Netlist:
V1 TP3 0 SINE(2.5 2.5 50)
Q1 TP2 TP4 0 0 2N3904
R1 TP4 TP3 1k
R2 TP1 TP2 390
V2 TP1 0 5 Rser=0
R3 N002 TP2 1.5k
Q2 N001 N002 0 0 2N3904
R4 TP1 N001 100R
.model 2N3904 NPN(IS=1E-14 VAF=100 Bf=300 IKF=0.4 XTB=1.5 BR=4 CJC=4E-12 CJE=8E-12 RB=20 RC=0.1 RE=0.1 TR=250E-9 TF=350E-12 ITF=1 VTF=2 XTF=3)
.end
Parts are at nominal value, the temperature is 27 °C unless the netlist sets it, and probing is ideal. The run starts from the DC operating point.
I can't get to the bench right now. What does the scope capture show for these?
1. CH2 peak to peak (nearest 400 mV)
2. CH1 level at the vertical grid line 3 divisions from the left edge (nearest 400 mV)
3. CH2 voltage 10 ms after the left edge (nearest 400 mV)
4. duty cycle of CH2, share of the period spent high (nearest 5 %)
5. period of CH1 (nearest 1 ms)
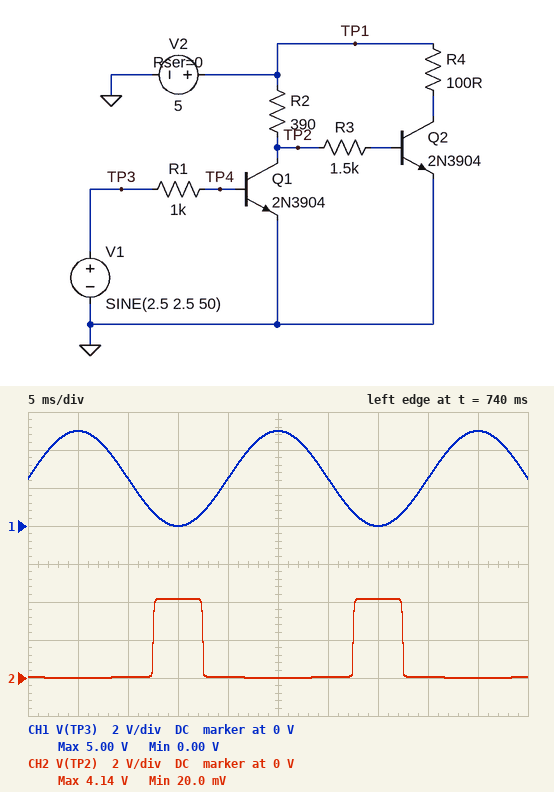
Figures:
4.0 V
0 V
0 V
25 %
20 ms
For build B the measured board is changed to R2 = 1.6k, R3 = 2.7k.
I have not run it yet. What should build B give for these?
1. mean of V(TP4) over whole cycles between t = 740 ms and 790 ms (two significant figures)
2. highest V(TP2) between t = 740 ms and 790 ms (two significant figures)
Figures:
640 mV
3.4 V
